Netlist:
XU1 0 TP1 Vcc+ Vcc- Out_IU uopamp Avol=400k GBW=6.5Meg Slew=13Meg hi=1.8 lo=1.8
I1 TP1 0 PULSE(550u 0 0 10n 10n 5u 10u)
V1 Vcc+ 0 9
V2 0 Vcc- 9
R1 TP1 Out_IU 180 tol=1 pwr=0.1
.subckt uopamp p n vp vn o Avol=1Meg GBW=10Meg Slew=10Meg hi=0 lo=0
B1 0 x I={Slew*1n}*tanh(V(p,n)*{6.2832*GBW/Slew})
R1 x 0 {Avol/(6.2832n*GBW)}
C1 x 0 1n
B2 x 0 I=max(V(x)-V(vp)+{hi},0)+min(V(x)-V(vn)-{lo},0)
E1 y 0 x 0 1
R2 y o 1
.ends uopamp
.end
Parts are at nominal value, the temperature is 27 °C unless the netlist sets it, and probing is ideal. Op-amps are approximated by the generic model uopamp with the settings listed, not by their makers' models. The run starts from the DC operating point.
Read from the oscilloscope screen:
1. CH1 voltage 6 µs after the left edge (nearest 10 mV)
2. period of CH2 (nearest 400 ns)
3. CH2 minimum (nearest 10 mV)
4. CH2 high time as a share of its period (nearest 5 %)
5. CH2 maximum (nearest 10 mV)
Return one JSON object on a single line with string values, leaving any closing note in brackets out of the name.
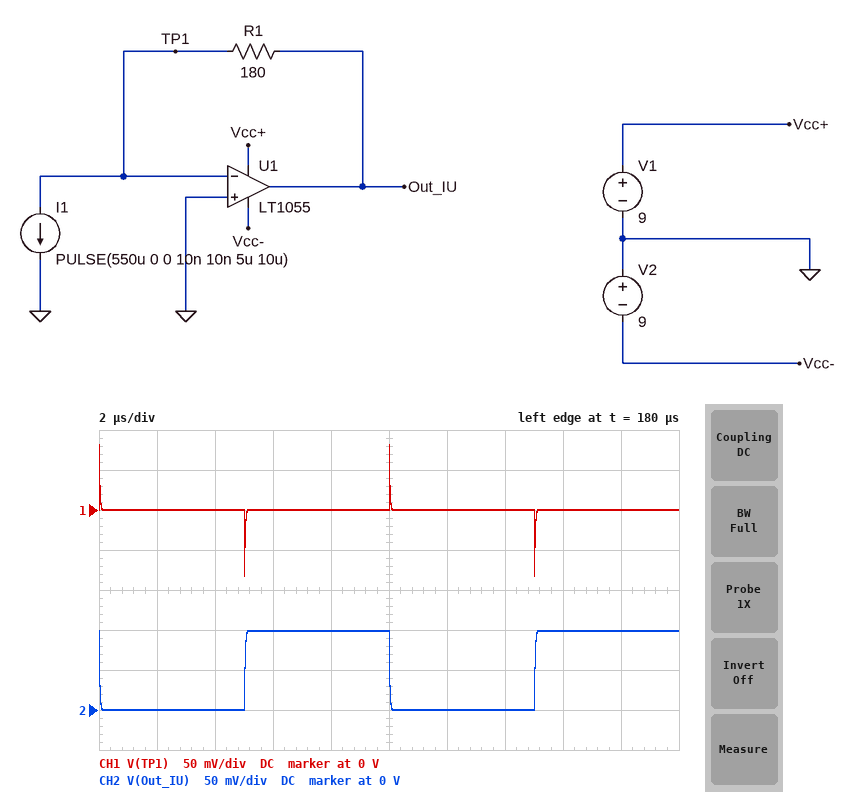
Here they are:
{"CH1 voltage 6 µs after the left edge": "0 V", "period of CH2": "10.0 µs", "CH2 minimum": "0 V", "CH2 high time as a share of its period": "50 %", "CH2 maximum": "100 mV"}
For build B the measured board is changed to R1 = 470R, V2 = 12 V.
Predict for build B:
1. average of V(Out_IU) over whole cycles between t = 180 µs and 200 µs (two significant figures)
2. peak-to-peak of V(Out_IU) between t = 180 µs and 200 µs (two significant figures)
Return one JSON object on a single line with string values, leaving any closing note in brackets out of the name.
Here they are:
{"average of V(Out_IU) over whole cycles between t = 180 µs and 200 µs": "130 mV", "peak-to-peak of V(Out_IU) between t = 180 µs and 200 µs": "260 mV"}
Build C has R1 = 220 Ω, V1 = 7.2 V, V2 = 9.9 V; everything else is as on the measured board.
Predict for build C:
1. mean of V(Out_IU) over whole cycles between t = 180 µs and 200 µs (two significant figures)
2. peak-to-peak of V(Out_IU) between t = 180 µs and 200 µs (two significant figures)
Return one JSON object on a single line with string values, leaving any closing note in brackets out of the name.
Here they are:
{"mean of V(Out_IU) over whole cycles between t = 180 µs and 200 µs": "60 mV", "peak-to-peak of V(Out_IU) between t = 180 µs and 200 µs": "120 mV"}
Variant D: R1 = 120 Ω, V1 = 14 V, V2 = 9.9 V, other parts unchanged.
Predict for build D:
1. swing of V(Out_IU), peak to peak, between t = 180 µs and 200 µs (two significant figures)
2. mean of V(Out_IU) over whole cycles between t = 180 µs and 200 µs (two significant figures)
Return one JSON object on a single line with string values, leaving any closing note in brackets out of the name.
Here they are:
{"swing of V(Out_IU), peak to peak, between t = 180 µs and 200 µs": "66 mV", "mean of V(Out_IU) over whole cycles between t = 180 µs and 200 µs": "33 mV"}
